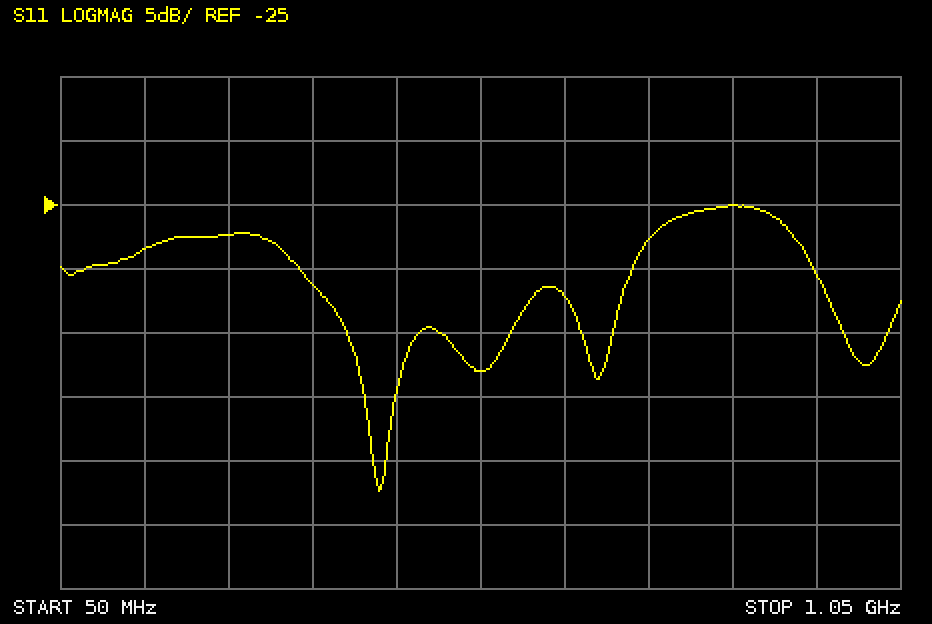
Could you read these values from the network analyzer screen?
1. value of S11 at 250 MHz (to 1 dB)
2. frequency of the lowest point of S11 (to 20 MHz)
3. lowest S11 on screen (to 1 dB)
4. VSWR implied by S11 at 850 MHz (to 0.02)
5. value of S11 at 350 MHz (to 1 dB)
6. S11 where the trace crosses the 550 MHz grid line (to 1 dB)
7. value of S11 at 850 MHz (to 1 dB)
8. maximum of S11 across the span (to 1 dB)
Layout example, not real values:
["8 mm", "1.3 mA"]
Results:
["-27 dB", "420 MHz", "-47 dB", "1.12", "-31 dB", "-38 dB", "-25 dB", "-25 dB"]
